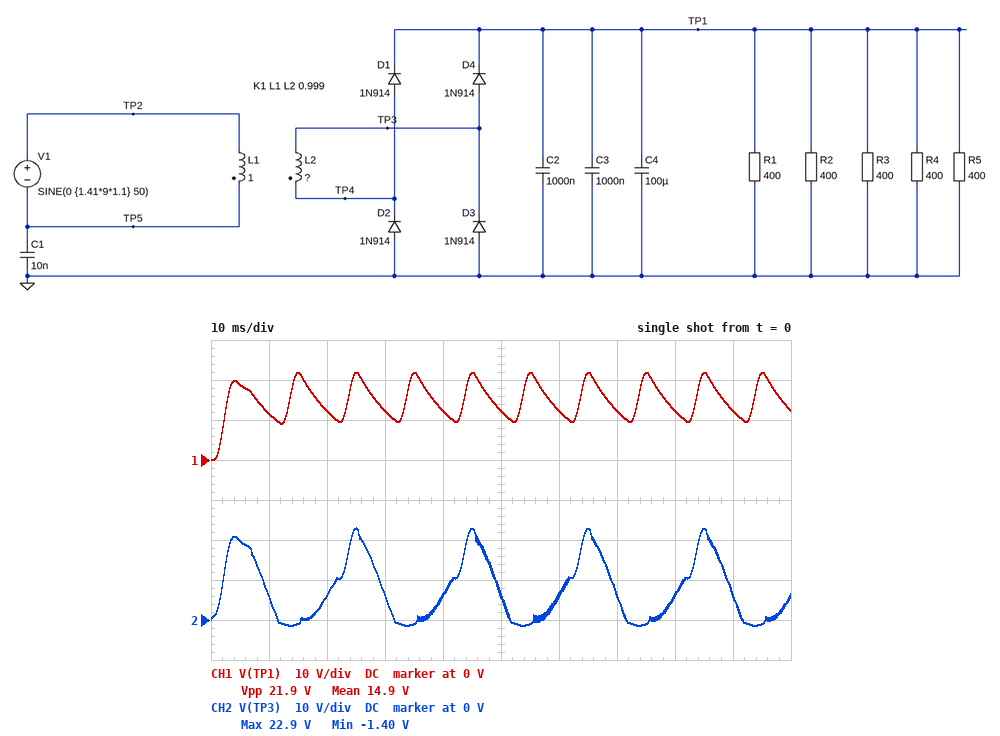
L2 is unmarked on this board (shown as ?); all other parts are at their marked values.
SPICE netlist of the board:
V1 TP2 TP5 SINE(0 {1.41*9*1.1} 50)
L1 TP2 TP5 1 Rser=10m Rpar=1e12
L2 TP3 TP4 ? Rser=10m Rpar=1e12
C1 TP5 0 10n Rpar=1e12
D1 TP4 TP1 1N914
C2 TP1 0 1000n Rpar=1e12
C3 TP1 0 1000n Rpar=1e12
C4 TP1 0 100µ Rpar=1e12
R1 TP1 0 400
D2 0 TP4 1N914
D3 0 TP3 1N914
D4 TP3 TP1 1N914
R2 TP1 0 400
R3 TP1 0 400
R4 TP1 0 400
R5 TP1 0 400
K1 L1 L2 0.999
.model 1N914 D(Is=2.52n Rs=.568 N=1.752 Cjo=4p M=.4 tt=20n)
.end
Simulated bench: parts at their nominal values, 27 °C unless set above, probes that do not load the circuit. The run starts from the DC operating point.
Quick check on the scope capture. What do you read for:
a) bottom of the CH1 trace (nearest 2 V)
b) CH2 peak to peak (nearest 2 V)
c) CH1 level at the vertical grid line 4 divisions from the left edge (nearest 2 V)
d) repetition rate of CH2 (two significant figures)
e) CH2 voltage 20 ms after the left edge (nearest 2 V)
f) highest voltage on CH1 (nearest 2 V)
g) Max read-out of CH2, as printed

0 V
24 V
12 V
50 Hz
6 V
22 V
22.9 V
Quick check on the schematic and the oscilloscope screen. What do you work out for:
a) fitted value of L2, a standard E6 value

2.2 H
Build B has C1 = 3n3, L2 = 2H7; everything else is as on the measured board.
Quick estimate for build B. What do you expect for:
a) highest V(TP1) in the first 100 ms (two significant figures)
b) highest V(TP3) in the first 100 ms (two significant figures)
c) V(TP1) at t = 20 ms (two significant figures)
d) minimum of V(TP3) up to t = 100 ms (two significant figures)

25 V
26 V
14 V
-1.5 V
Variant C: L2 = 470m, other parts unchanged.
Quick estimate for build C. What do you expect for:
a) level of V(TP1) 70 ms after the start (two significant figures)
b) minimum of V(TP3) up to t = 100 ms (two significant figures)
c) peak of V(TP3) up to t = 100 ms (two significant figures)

4.7 V
-1.1 V
8.8 V
